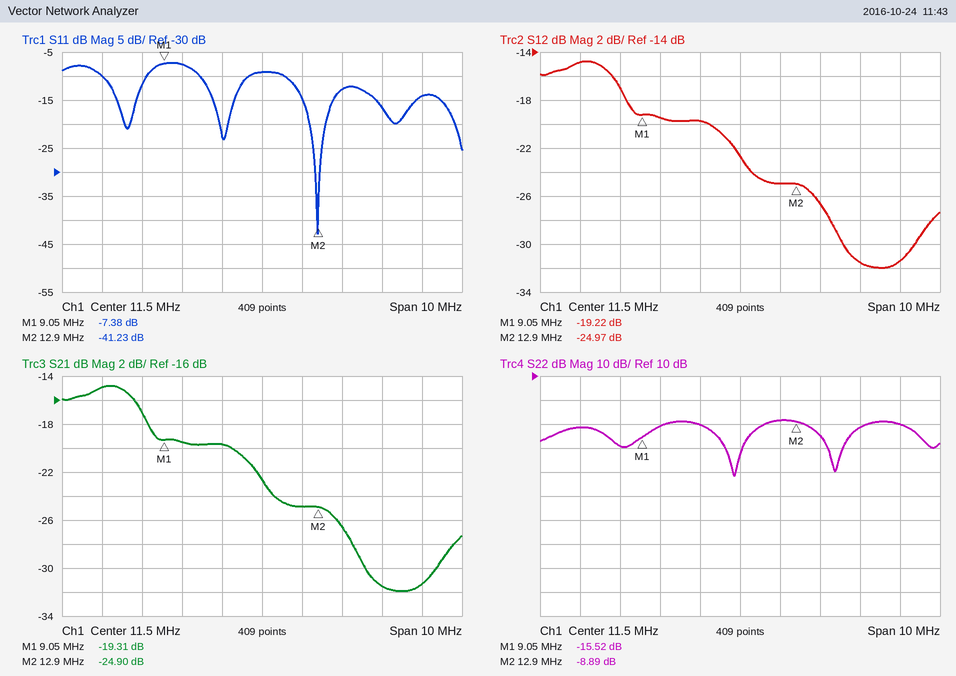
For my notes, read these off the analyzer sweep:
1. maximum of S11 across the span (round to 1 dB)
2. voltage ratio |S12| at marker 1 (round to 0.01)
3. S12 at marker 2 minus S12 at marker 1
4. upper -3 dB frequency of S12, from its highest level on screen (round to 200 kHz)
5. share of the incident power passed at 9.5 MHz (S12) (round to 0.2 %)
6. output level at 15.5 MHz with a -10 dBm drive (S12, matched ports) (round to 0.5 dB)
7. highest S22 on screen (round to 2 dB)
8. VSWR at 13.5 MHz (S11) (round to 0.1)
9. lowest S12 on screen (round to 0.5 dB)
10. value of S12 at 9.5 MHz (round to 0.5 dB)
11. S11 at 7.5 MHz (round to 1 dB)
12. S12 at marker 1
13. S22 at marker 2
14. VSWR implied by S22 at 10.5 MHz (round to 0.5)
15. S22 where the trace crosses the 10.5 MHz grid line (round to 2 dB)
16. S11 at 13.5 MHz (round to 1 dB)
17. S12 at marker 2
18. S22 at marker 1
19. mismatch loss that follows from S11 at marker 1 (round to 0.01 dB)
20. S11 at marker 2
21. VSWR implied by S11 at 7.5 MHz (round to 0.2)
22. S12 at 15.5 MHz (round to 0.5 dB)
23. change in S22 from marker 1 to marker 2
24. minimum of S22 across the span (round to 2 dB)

-7 dB
0.11
-5.75 dB
8.6 MHz
1.2 %
-41.5 dBm
-8 dB
1.6
-32.0 dB
-19.5 dB
-10 dB
-19.22 dB
-8.89 dB
2.0
-10 dB
-13 dB
-24.97 dB
-15.52 dB
0.88 dB
-41.23 dB
2.0
-31.5 dB
6.63 dB
-32 dB
